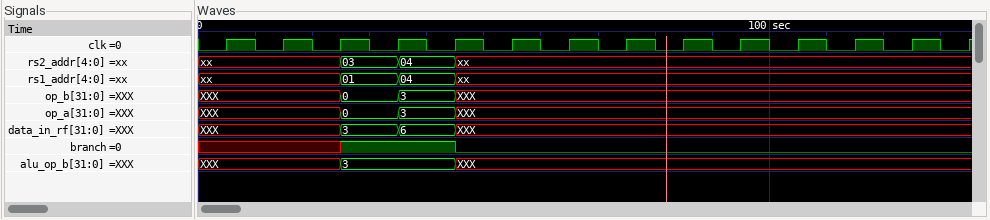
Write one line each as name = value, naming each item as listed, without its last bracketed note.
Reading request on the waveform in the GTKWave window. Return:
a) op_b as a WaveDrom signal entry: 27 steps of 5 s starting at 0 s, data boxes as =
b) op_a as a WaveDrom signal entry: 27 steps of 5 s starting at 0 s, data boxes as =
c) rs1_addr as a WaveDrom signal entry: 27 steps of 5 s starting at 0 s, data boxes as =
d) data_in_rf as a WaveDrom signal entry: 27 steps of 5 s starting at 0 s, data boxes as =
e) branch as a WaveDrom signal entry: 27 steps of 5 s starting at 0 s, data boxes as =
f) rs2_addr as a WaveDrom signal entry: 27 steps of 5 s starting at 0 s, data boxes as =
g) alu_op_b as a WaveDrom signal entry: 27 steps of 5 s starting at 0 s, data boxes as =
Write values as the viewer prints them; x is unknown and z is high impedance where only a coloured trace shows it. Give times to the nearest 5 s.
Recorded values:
op_b as a WaveDrom signal entry: 27 steps of 5 s starting at 0 s, data boxes as = = {name: 'op_b', wave: 'x....=.=.x.................', data: '0 3'}
op_a as a WaveDrom signal entry: 27 steps of 5 s starting at 0 s, data boxes as = = {name: 'op_a', wave: 'x....=.=.x.................', data: '0 3'}
rs1_addr as a WaveDrom signal entry: 27 steps of 5 s starting at 0 s, data boxes as = = {name: 'rs1_addr', wave: 'x....=.=.x.................', data: '01 04'}
data_in_rf as a WaveDrom signal entry: 27 steps of 5 s starting at 0 s, data boxes as = = {name: 'data_in_rf', wave: 'x....=.=.x.................', data: '3 6'}
branch as a WaveDrom signal entry: 27 steps of 5 s starting at 0 s, data boxes as = = {name: 'branch', wave: 'x....1...0.................'}
rs2_addr as a WaveDrom signal entry: 27 steps of 5 s starting at 0 s, data boxes as = = {name: 'rs2_addr', wave: 'x....=.=.x.................', data: '03 04'}
alu_op_b as a WaveDrom signal entry: 27 steps of 5 s starting at 0 s, data boxes as = = {name: 'alu_op_b', wave: 'x....=...x.................', data: '3'}
